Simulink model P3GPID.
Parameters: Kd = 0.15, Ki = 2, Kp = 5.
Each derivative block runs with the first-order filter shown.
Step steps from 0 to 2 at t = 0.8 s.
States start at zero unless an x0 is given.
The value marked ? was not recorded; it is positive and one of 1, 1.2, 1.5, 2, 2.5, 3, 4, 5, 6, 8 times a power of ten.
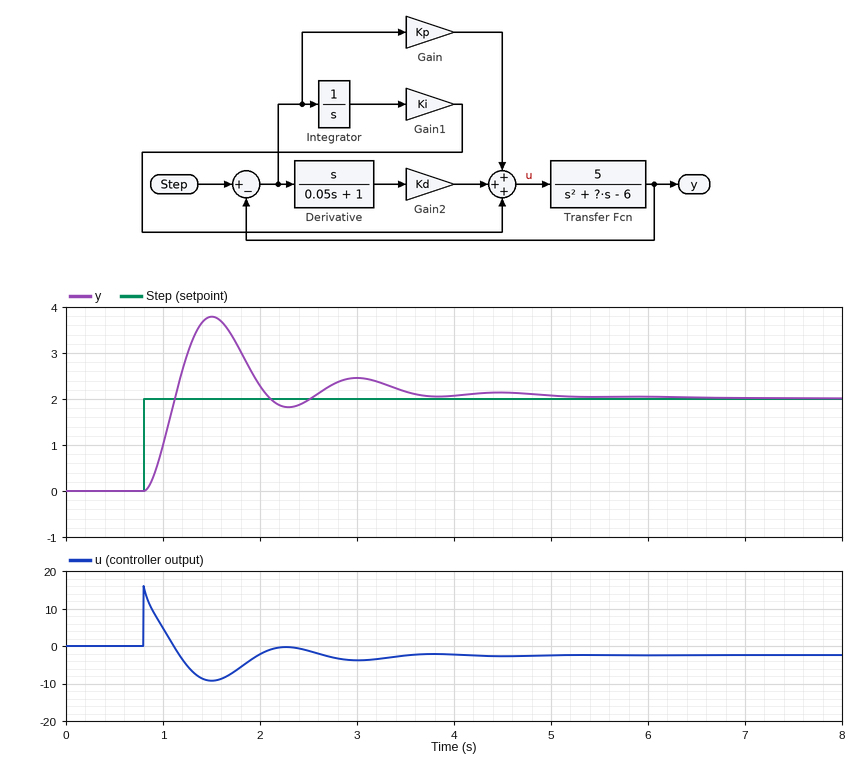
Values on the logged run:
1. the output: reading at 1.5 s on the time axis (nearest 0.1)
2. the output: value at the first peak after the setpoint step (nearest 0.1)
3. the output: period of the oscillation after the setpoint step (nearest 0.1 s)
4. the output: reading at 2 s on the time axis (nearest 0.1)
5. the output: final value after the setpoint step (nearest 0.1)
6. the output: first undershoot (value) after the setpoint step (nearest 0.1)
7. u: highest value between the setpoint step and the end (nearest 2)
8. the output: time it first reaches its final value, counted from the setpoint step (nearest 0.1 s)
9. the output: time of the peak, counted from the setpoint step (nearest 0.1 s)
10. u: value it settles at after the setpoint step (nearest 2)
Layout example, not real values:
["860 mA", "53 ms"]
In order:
["3.8", "3.8", "1.5 s", "2.3", "2.0", "1.8", "16", "0.3 s", "0.7 s", "-2"]
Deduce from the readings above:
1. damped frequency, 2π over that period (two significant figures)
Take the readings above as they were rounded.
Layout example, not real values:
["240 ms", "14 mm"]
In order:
["4.2 rad/s"]
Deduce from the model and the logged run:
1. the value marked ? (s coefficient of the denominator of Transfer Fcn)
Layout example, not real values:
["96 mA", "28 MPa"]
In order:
["2"]
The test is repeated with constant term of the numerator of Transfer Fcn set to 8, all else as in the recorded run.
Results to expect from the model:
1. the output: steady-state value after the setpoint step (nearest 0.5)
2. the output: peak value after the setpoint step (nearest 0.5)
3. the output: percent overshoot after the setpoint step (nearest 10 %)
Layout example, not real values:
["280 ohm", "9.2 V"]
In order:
["2.0", "3.5", "80 %"]
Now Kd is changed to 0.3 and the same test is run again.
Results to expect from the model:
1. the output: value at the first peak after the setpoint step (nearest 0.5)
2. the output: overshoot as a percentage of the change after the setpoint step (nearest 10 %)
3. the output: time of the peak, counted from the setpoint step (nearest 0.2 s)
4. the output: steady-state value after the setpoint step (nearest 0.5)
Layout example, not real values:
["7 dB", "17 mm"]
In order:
["3.5", "80 %", "0.6 s", "2.0"]
